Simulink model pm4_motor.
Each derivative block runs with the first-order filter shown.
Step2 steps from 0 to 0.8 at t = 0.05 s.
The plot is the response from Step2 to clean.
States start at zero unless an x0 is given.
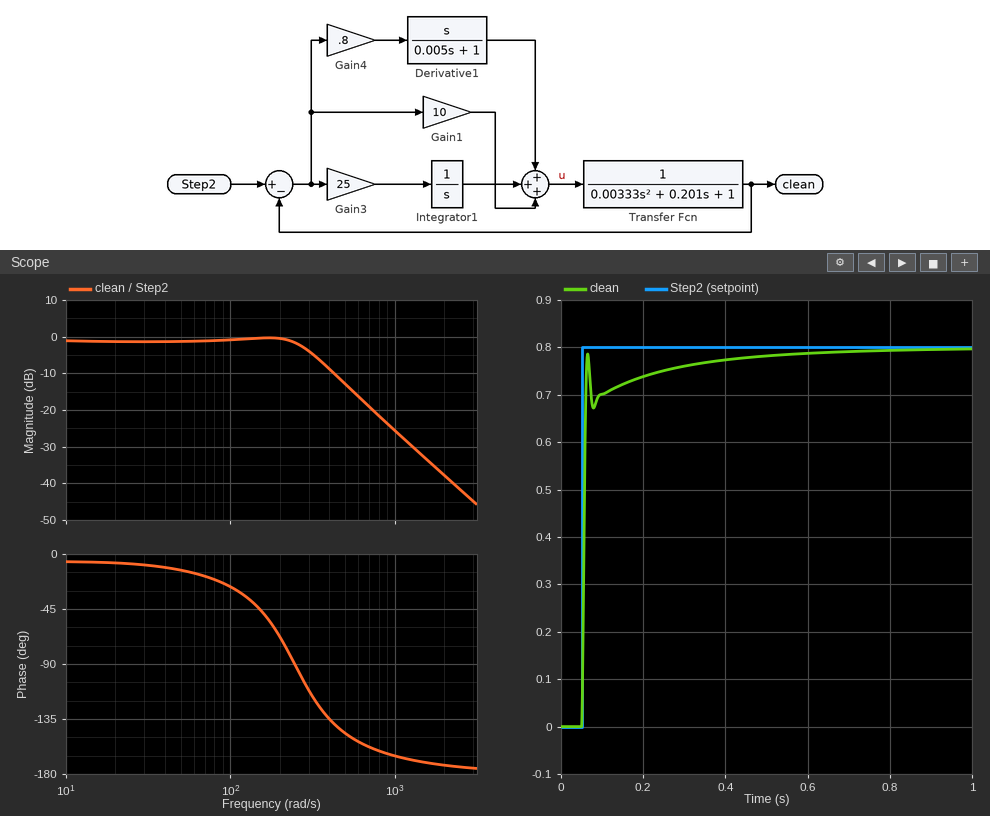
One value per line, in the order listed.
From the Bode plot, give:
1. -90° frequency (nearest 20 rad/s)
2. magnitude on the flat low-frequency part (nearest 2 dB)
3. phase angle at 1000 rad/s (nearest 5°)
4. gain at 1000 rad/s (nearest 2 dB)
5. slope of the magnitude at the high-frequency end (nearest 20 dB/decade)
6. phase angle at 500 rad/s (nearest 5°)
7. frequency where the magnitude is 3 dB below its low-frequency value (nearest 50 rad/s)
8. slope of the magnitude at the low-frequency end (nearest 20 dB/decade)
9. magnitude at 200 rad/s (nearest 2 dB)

240 rad/s
-2 dB
-165°
-26 dB
-40 dB/decade
-145°
300 rad/s
0 dB/decade
0 dB
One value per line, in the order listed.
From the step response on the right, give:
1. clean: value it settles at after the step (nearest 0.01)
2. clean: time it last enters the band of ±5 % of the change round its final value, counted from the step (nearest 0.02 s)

0.80
0.24 s
